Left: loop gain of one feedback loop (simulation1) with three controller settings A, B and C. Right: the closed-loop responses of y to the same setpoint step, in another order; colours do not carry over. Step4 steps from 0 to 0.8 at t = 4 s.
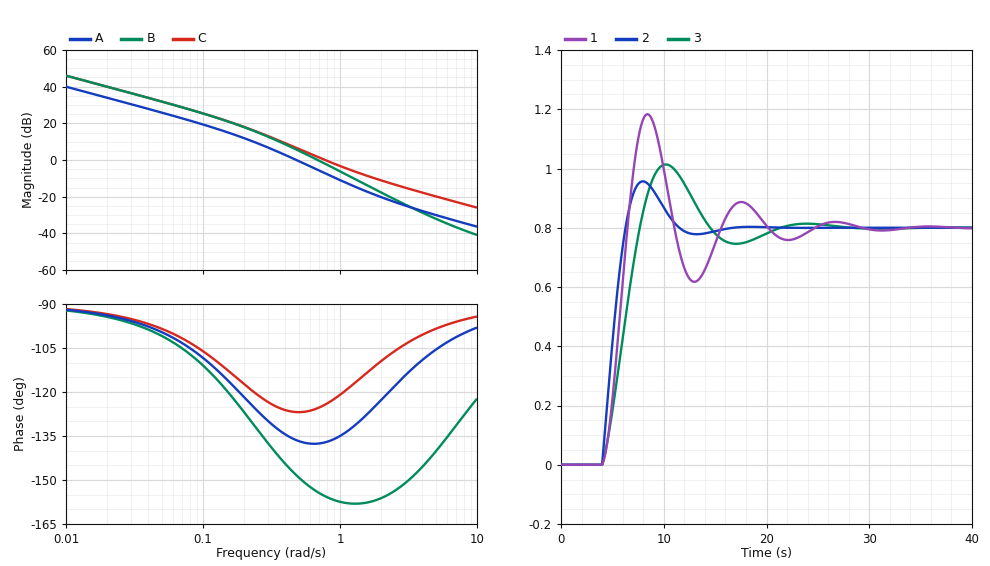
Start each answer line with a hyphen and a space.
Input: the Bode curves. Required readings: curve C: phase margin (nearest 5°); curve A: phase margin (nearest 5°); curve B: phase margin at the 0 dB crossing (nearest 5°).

- 55°
- 45°
- 25°
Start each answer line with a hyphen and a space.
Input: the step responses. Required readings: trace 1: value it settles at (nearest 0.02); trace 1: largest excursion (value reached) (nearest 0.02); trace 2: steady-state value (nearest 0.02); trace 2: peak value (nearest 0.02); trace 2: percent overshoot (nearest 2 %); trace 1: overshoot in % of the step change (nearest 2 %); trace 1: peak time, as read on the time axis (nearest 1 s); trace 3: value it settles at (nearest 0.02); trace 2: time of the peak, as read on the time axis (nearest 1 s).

- 0.80
- 1.18
- 0.80
- 0.96
- 20 %
- 48 %
- 8 s
- 0.80
- 8 s
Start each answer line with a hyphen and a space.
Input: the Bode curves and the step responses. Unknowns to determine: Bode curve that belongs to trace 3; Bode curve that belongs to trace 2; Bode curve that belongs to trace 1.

- A
- C
- B
